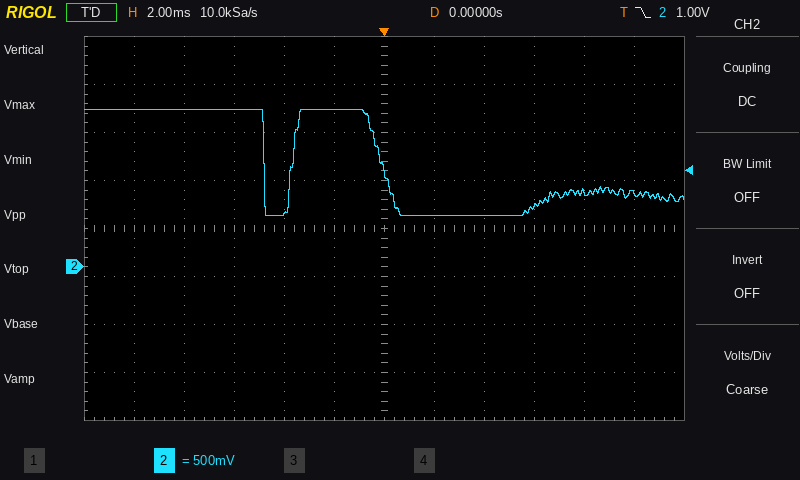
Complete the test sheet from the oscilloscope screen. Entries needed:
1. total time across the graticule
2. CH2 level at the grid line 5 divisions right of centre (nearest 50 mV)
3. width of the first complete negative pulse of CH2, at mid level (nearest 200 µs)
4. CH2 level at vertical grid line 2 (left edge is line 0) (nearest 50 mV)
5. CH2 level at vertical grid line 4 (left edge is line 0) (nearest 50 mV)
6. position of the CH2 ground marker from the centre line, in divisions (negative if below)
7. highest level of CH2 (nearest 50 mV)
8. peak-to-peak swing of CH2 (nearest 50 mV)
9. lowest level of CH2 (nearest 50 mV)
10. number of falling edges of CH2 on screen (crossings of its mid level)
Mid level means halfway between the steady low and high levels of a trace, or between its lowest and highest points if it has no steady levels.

24 ms
750 mV
1.2 ms
1.65 V
550 mV
-0.8 div
1.65 V
1.10 V
550 mV
2
